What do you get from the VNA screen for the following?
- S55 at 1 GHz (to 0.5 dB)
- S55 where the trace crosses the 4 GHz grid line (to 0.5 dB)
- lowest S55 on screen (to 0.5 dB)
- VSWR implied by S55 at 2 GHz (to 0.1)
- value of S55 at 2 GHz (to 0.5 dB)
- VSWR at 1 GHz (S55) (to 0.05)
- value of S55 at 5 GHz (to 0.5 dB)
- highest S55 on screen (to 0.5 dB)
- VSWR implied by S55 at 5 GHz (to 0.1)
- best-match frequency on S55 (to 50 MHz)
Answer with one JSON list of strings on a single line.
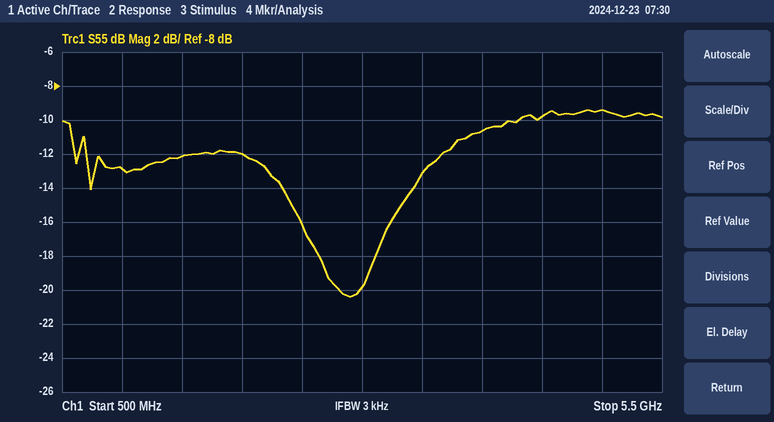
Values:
["-13.0 dB", "-10.5 dB", "-20.5 dB", "1.7", "-12.0 dB", "1.60", "-9.5 dB", "-9.5 dB", "2.0", "2.90 GHz"]
